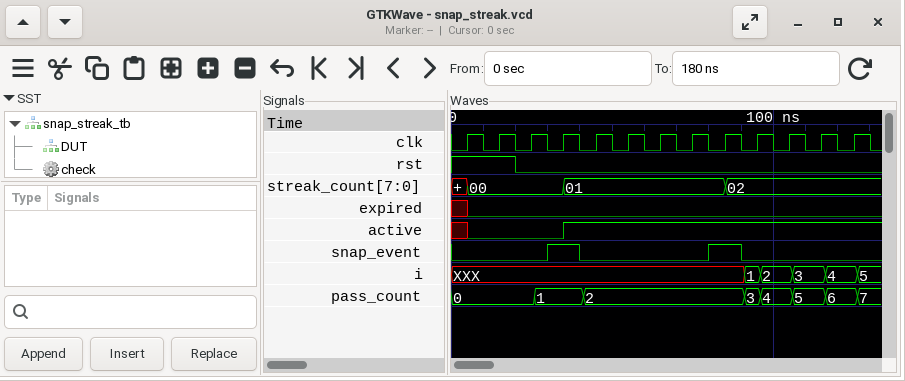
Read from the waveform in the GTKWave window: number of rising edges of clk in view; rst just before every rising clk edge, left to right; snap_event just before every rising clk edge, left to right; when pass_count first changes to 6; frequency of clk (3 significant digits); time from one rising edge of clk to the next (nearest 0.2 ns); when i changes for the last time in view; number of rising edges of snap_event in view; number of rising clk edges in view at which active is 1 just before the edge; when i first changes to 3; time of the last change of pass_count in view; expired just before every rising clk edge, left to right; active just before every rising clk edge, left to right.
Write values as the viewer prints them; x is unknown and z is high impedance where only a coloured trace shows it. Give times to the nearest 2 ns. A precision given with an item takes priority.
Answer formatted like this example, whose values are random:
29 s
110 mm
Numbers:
13
1 1 0 0 0 0 0 0 0 0 0 0 0
0 0 0 1 0 0 0 0 1 0 0 0 0
116 ns
100 MHz
10 ns
126 ns
2
9
106 ns
126 ns
x 0 0 0 0 0 0 0 0 0 0 0 0
x 0 0 0 1 1 1 1 1 1 1 1 1
